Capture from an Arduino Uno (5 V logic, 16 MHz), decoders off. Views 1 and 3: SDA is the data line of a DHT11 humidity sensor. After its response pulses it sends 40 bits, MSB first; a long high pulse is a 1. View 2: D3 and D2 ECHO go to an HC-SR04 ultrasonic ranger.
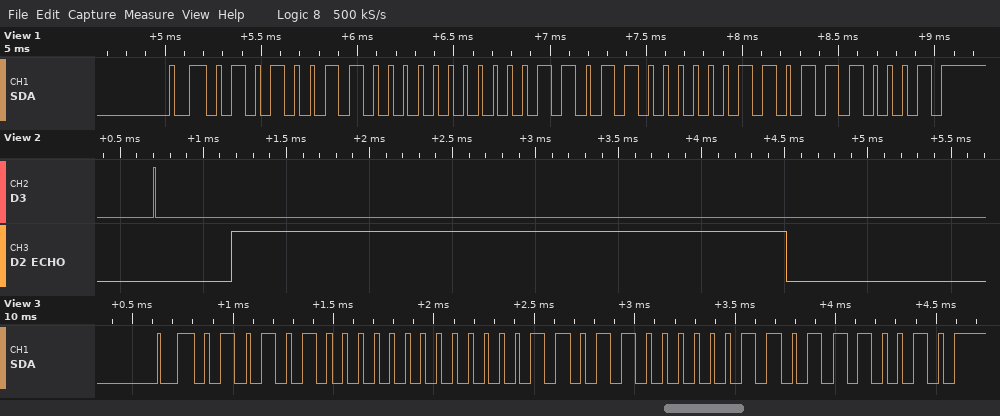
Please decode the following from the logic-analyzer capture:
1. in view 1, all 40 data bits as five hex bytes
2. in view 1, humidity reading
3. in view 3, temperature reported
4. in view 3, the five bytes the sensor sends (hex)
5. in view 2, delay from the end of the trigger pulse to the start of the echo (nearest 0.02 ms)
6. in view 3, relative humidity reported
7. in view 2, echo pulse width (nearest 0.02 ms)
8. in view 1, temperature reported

53 00 1B 03 71
83 %
27.3 °C
54 00 1B 03 72
0.46 ms
84 %
3.34 ms
27.3 °C
